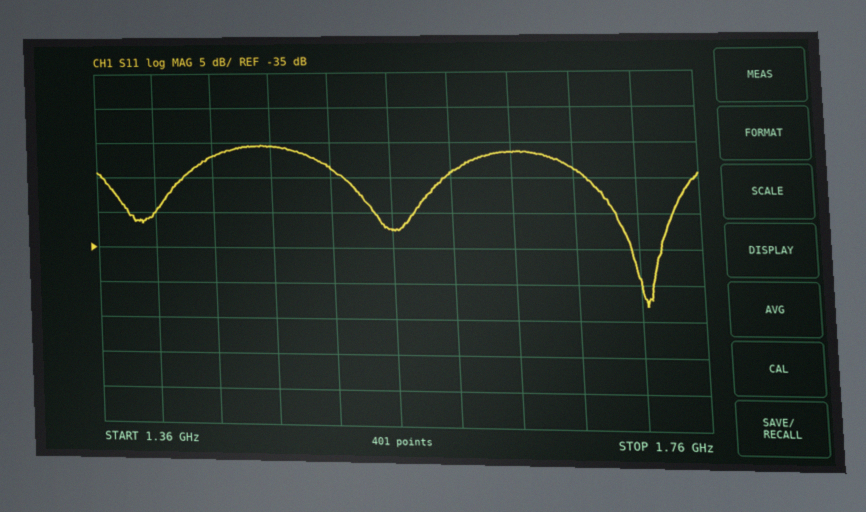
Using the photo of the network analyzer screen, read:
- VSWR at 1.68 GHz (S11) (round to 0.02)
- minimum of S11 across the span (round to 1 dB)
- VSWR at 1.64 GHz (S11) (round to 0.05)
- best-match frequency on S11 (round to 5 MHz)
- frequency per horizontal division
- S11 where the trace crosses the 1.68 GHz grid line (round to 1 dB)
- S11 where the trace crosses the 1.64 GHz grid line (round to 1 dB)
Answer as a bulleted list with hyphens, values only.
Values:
- 1.14
- -43 dB
- 1.20
- 1.725 GHz
- 40 MHz
- -24 dB
- -21 dB
